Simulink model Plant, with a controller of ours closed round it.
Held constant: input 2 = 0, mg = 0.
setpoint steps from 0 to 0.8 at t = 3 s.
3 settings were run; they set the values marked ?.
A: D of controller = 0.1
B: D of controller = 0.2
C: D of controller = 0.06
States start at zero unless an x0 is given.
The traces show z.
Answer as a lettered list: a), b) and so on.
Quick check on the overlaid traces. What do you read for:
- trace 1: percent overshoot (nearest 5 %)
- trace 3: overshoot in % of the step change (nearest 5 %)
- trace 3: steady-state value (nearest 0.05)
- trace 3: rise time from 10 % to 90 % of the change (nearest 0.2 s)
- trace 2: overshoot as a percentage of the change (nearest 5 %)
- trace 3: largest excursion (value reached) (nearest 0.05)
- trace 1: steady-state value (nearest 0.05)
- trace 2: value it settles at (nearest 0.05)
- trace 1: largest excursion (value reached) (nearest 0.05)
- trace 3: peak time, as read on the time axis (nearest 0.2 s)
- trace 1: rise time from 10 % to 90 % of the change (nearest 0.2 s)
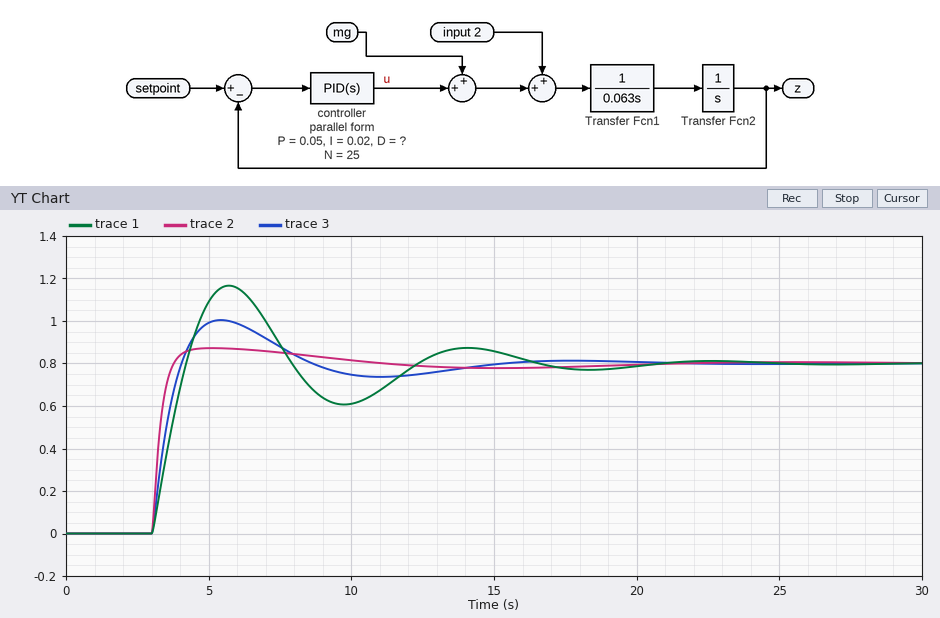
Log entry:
a) 45 %
b) 25 %
c) 0.80
d) 0.8 s
e) 10 %
f) 1.00
g) 0.80
h) 0.80
i) 1.15
j) 5.4 s
k) 1.0 s
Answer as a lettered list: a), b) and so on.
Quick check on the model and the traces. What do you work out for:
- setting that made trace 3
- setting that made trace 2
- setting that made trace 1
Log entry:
a) A
b) B
c) C
